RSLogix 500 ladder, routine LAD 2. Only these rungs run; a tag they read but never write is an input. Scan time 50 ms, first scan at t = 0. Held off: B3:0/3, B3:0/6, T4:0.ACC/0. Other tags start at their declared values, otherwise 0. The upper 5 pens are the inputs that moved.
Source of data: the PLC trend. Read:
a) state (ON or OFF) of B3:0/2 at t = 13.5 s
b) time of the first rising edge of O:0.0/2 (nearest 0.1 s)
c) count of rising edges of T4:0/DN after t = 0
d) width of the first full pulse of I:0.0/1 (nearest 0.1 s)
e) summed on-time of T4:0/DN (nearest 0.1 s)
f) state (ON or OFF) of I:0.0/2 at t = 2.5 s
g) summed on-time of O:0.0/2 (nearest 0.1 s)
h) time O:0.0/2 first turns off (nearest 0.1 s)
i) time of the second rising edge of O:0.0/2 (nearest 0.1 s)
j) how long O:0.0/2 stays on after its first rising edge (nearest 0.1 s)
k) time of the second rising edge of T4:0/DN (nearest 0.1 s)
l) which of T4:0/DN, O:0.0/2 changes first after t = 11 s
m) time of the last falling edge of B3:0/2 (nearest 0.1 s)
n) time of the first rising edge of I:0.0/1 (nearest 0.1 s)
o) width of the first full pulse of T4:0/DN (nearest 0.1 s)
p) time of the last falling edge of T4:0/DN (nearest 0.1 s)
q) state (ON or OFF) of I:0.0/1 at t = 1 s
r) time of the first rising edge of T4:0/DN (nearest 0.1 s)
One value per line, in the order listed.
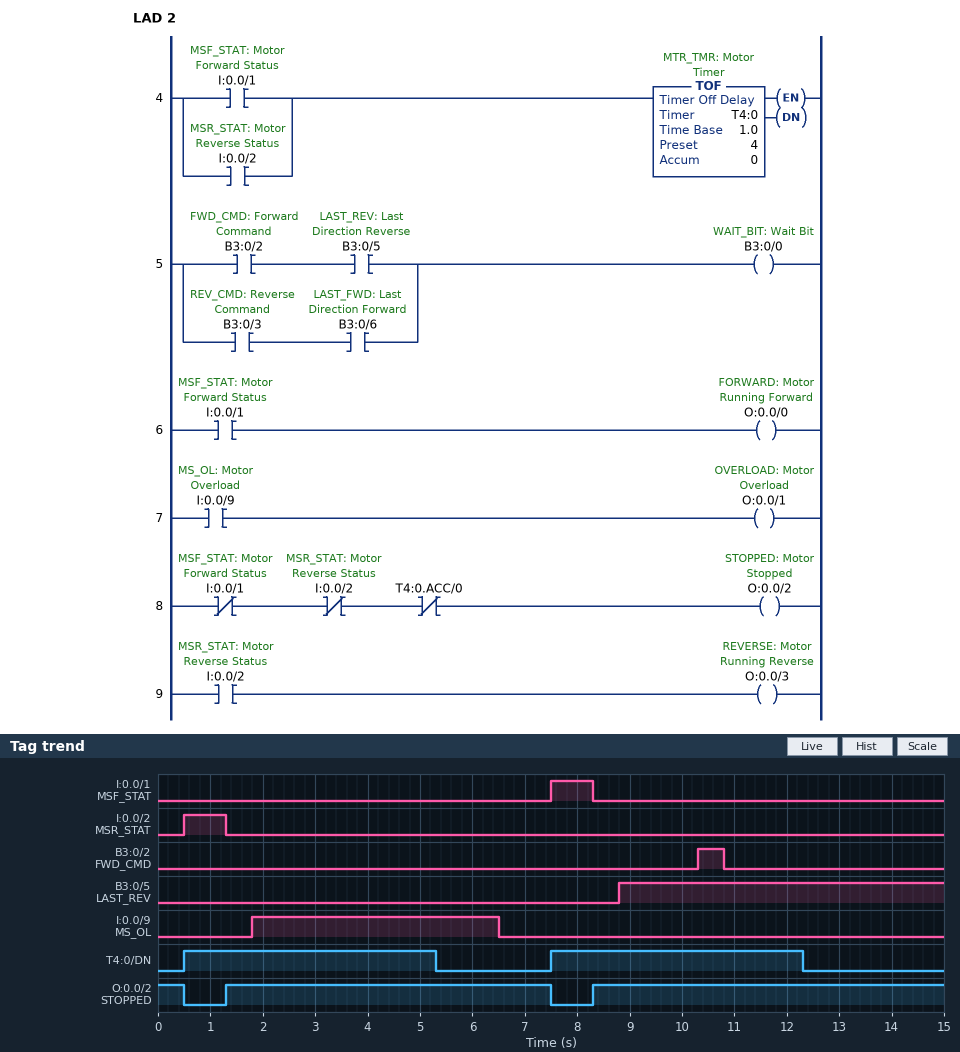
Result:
OFF
1.3 s
2
0.8 s
9.6 s
OFF
13.4 s
0.5 s
8.3 s
6.2 s
7.5 s
T4:0/DN
10.8 s
7.5 s
4.8 s
12.3 s
OFF
0.5 s
